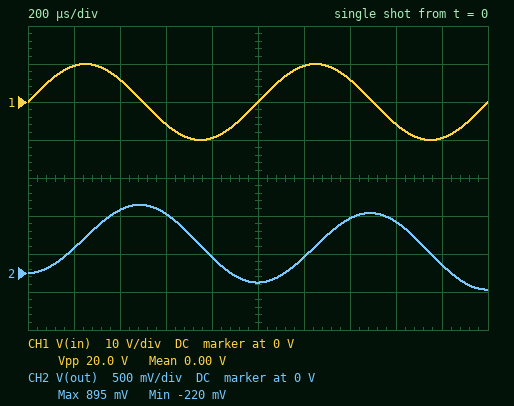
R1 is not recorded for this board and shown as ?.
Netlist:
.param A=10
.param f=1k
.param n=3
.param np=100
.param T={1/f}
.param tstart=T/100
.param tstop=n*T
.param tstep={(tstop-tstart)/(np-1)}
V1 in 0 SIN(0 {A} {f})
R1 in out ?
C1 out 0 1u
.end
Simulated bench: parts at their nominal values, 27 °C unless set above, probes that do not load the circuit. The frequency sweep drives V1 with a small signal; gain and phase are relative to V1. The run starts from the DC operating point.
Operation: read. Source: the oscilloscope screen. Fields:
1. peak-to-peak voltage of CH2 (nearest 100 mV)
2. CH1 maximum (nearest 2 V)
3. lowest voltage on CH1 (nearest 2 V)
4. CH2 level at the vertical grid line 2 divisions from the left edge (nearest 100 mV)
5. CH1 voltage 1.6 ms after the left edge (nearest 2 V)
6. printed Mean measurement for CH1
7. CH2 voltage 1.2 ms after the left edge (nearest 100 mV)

1.1 V
10 V
-10 V
800 mV
-6 V
0.00 V
200 mV
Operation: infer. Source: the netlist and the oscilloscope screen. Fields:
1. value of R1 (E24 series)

3.3 kΩ
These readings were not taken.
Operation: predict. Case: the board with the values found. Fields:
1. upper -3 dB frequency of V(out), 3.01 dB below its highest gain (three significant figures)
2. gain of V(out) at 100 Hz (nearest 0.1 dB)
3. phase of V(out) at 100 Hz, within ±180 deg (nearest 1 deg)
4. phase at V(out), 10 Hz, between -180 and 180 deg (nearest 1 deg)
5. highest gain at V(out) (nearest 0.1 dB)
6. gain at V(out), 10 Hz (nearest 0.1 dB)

48.2 Hz
-7.2 dB
-64 deg
-12 deg
0 dB
-0.2 dB
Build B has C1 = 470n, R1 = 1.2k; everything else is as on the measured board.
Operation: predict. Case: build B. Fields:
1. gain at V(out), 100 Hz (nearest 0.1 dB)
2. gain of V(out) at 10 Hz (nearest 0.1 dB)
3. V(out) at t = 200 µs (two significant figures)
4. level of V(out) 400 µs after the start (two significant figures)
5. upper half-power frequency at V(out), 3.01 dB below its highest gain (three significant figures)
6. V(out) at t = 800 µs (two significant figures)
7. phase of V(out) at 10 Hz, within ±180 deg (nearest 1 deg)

-0.5 dB
0 dB
1.7 V
3.8 V
282 Hz
-880 mV
-2 deg
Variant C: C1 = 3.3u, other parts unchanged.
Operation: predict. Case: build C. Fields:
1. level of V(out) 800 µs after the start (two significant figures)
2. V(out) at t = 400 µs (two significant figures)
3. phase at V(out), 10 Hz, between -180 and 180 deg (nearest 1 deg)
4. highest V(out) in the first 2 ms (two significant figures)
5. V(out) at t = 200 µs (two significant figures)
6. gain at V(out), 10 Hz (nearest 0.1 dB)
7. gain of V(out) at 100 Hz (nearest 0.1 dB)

89 mV
260 mV
-34 deg
290 mV
100 mV
-1.7 dB
-16.8 dB
